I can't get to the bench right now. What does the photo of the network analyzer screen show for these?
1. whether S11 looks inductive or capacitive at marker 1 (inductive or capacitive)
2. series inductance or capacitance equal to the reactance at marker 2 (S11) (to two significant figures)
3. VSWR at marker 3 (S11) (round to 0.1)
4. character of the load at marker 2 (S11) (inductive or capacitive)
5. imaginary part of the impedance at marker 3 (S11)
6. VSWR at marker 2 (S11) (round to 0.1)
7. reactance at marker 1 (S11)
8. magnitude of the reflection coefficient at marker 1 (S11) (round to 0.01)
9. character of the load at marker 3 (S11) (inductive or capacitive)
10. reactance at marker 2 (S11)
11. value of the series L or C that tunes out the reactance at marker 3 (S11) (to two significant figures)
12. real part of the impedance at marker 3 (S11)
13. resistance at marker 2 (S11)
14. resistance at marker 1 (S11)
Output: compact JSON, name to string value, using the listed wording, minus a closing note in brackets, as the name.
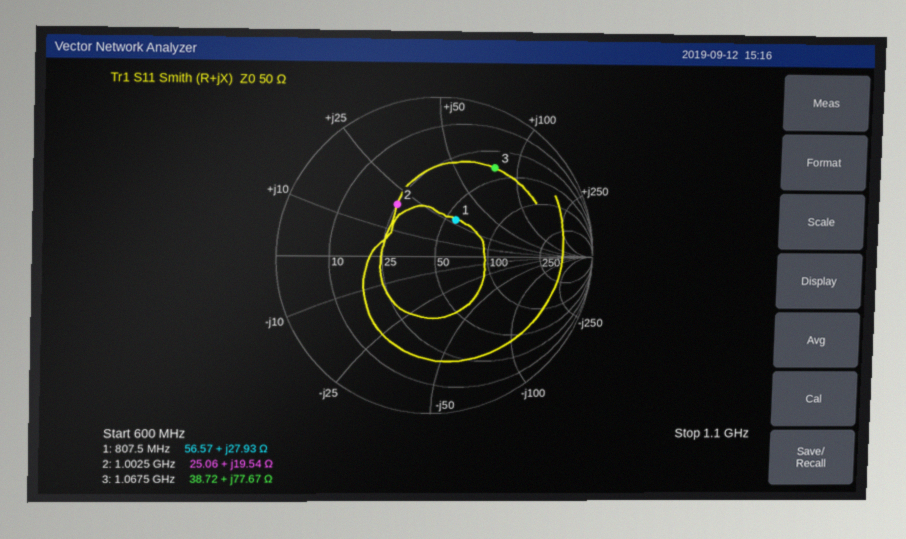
{"whether S11 looks inductive or capacitive at marker 1": "inductive", "series inductance or capacitance equal to the reactance at marker 2 (S11)": "3.1 nH", "VSWR at marker 3 (S11)": "5.0", "character of the load at marker 2 (S11)": "inductive", "imaginary part of the impedance at marker 3": "+77.67 Ω", "VSWR at marker 2 (S11)": "2.4", "reactance at marker 1": "+27.93 Ω", "magnitude of the reflection coefficient at marker 1 (S11)": "0.26", "character of the load at marker 3 (S11)": "inductive", "reactance at marker 2": "+19.54 Ω", "value of the series L or C that tunes out the reactance at marker 3 (S11)": "1.9 pF", "real part of the impedance at marker 3": "38.72 Ω", "resistance at marker 2": "25.06 Ω", "resistance at marker 1": "56.57 Ω"}
